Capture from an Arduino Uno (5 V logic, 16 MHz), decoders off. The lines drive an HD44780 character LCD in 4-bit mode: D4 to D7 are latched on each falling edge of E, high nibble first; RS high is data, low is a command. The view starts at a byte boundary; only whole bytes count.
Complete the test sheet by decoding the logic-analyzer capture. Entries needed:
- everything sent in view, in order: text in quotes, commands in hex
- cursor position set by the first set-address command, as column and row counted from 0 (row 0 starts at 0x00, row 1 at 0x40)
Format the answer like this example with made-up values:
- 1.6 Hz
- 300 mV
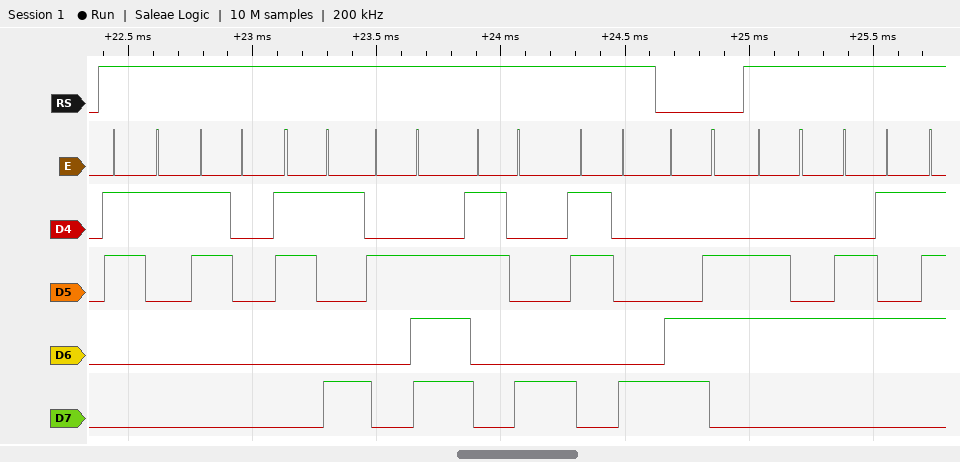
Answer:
- "109.88" 0xC6 "de"
- column 6, row 1
